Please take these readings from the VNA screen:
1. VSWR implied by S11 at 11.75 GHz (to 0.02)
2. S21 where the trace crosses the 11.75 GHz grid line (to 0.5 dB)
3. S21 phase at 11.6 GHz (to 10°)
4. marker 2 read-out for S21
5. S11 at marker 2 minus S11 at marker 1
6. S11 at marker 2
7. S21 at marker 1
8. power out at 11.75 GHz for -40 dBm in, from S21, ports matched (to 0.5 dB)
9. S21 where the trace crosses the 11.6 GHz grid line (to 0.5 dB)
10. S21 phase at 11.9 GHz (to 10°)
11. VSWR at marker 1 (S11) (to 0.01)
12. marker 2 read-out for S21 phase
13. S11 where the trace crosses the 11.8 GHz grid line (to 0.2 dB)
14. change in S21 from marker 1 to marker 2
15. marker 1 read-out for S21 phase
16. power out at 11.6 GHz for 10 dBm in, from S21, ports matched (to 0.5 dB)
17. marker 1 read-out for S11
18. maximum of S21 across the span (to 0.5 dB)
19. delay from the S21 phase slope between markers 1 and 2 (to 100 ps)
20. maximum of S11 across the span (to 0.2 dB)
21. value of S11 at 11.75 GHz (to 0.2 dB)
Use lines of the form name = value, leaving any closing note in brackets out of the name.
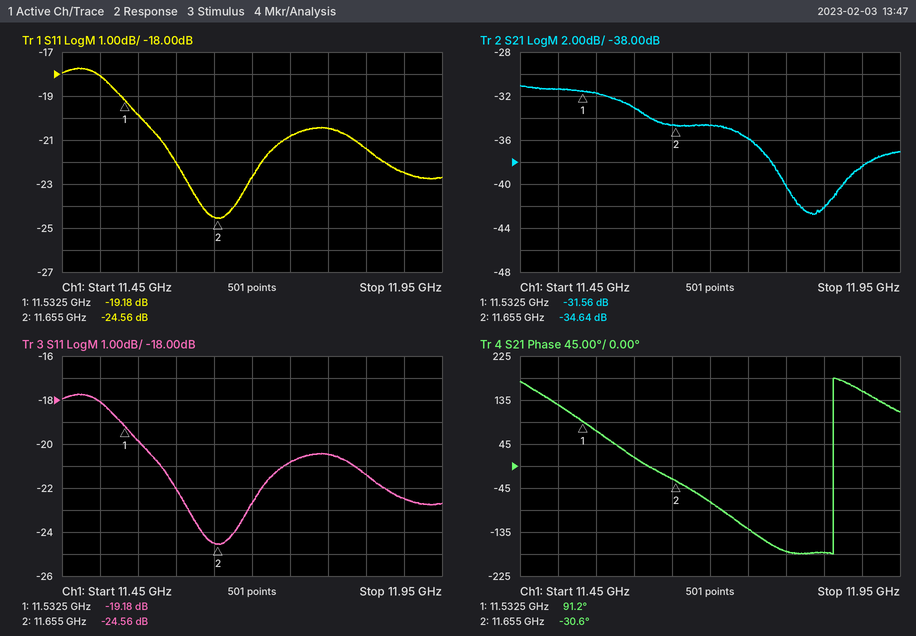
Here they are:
VSWR implied by S11 at 11.75 GHz = 1.20
S21 where the trace crosses the 11.75 GHz grid line = -36.0 dB
S21 phase at 11.6 GHz = 20°
marker 2 read-out for S21 = -34.64 dB
S11 at marker 2 minus S11 at marker 1 = -5.38 dB
S11 at marker 2 = -24.56 dB
S21 at marker 1 = -31.56 dB
power out at 11.75 GHz for -40 dBm in, from S21, ports matched = -76.0 dBm
S21 where the trace crosses the 11.6 GHz grid line = -33.0 dB
S21 phase at 11.9 GHz = 150°
VSWR at marker 1 (S11) = 1.25
marker 2 read-out for S21 phase = -30.6°
S11 where the trace crosses the 11.8 GHz grid line = -20.4 dB
change in S21 from marker 1 to marker 2 = -3.08 dB
marker 1 read-out for S21 phase = 91.2°
power out at 11.6 GHz for 10 dBm in, from S21, ports matched = -23.0 dBm
marker 1 read-out for S11 = -19.18 dB
maximum of S21 across the span = -31.0 dB
delay from the S21 phase slope between markers 1 and 2 = 2.8 ns
maximum of S11 across the span = -17.8 dB
value of S11 at 11.75 GHz = -20.8 dB
